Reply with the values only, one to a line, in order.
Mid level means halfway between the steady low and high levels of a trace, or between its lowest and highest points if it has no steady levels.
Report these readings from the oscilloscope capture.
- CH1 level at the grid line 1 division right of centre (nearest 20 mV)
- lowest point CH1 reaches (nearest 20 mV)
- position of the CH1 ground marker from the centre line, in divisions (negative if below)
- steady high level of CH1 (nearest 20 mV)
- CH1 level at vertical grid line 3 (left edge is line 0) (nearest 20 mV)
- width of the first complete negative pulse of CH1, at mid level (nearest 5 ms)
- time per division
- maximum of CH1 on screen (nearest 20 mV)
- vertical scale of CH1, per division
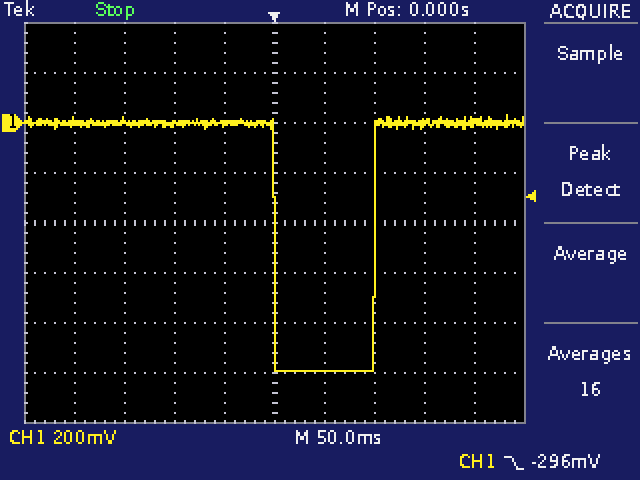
-1.00 V
-1.00 V
+2.0 div
0 mV
0 mV
100 ms
50 ms
40 mV
200 mV
